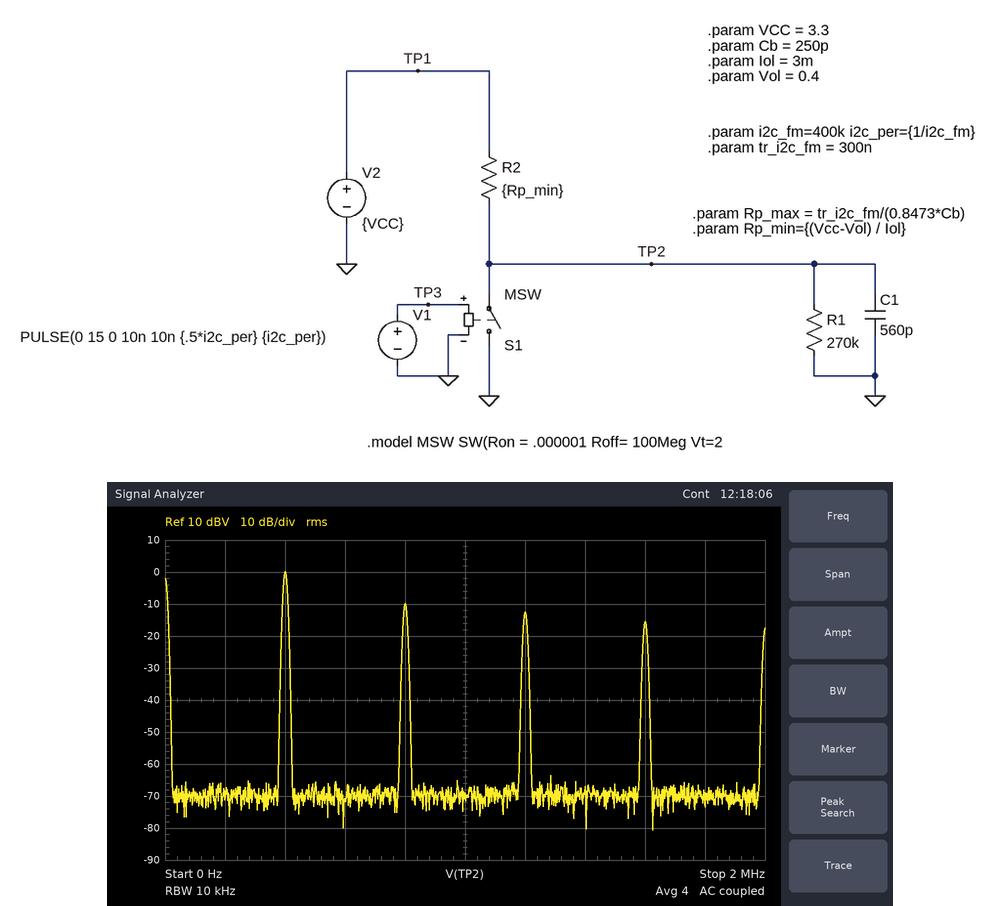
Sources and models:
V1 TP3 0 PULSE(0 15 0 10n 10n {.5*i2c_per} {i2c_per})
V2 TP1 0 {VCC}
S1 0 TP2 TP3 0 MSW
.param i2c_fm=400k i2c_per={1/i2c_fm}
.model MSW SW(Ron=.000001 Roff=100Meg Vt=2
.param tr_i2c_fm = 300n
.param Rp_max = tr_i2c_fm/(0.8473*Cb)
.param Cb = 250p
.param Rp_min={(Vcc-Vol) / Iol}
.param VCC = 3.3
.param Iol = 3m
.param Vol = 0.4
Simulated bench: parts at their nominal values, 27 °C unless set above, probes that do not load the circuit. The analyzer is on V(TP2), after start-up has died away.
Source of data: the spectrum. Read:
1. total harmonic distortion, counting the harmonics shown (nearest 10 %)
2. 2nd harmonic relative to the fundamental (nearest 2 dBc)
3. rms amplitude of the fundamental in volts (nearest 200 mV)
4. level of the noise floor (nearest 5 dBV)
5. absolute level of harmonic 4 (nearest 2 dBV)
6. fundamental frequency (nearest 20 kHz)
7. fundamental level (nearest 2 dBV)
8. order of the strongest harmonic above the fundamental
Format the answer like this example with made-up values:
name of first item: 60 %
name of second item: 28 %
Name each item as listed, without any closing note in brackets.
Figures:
total harmonic distortion, counting the harmonics shown: 40 %
2nd harmonic relative to the fundamental: -10 dBc
rms amplitude of the fundamental in volts: 1.0 V
level of the noise floor: -70 dBV
absolute level of harmonic 4: -16 dBV
fundamental frequency: 400 kHz
fundamental level: 0 dBV
order of the strongest harmonic above the fundamental: 2
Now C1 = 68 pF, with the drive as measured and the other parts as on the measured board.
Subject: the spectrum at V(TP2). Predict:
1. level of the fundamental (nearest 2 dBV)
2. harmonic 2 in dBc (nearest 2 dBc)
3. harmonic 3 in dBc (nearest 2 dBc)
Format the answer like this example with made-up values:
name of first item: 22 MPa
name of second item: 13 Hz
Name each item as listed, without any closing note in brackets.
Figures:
level of the fundamental: 4 dBV
harmonic 2 in dBc: -20 dBc
harmonic 3 in dBc: -10 dBc
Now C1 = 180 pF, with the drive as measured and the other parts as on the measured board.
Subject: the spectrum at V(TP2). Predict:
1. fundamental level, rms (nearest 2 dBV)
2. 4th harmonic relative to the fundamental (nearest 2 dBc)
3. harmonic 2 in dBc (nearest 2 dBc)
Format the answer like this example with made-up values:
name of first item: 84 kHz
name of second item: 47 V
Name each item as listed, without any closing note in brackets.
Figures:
fundamental level, rms: 2 dBV
4th harmonic relative to the fundamental: -18 dBc
harmonic 2 in dBc: -14 dBc
